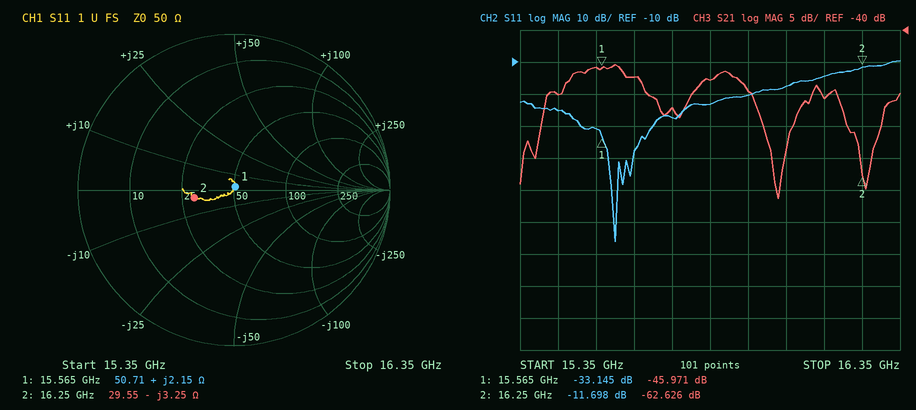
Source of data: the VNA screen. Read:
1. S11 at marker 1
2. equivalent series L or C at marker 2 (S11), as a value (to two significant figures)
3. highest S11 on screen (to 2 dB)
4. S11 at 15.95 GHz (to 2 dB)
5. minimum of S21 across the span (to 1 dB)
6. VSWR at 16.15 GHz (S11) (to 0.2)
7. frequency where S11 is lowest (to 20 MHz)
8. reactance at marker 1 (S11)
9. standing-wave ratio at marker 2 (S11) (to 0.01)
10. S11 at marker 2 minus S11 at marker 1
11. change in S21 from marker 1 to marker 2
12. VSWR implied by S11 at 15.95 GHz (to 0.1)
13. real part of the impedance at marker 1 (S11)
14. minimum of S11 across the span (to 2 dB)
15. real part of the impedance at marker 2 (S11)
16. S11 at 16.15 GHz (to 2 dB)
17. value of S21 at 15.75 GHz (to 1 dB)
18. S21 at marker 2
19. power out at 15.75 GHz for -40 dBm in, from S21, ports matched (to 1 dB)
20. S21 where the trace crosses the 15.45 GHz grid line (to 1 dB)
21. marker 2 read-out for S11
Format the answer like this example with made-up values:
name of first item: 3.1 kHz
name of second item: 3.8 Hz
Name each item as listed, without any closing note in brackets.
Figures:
S11 at marker 1: -33.145 dB
equivalent series L or C at marker 2 (S11), as a value: 3.0 pF
highest S11 on screen: -10 dB
S11 at 15.95 GHz: -20 dB
minimum of S21 across the span: -66 dB
VSWR at 16.15 GHz (S11): 1.4
frequency where S11 is lowest: 15.60 GHz
reactance at marker 1: +2.15 Ω
standing-wave ratio at marker 2 (S11): 1.70
S11 at marker 2 minus S11 at marker 1: 21.447 dB
change in S21 from marker 1 to marker 2: -16.655 dB
VSWR implied by S11 at 15.95 GHz: 1.2
real part of the impedance at marker 1: 50.71 Ω
minimum of S11 across the span: -66 dB
real part of the impedance at marker 2: 29.55 Ω
S11 at 16.15 GHz: -14 dB
value of S21 at 15.75 GHz: -52 dB
S21 at marker 2: -62.626 dB
power out at 15.75 GHz for -40 dBm in, from S21, ports matched: -92 dBm
S21 where the trace crosses the 15.45 GHz grid line: -50 dB
marker 2 read-out for S11: -11.698 dB
